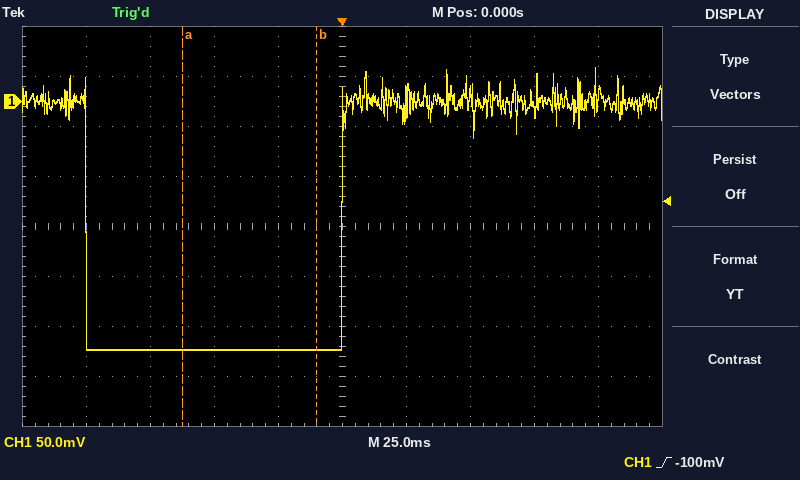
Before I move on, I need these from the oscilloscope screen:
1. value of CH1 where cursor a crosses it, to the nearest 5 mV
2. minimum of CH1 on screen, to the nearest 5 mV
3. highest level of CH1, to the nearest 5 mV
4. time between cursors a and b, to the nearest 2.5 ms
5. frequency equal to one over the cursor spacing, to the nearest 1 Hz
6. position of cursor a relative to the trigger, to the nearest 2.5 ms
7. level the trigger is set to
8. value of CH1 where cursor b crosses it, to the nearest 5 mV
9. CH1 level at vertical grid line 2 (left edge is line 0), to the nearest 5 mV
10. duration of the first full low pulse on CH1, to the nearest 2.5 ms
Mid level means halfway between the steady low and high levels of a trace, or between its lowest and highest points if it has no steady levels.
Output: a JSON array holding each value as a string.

["-250 mV", "-250 mV", "35 mV", "52.5 ms", "19 Hz", "-62.5 ms", "-100 mV", "-250 mV", "-250 mV", "100.0 ms"]
